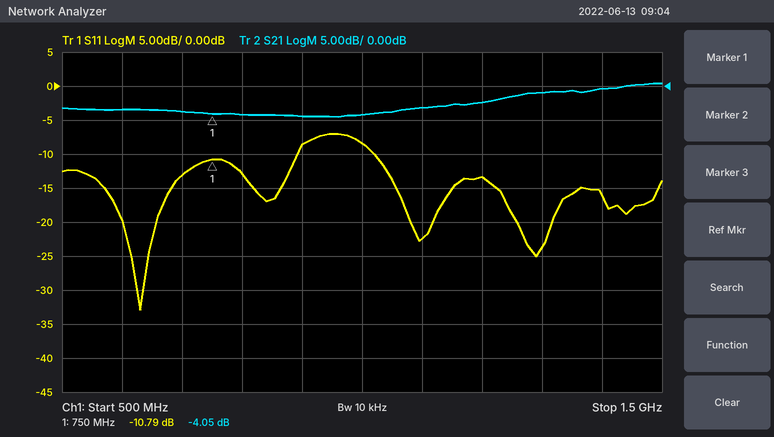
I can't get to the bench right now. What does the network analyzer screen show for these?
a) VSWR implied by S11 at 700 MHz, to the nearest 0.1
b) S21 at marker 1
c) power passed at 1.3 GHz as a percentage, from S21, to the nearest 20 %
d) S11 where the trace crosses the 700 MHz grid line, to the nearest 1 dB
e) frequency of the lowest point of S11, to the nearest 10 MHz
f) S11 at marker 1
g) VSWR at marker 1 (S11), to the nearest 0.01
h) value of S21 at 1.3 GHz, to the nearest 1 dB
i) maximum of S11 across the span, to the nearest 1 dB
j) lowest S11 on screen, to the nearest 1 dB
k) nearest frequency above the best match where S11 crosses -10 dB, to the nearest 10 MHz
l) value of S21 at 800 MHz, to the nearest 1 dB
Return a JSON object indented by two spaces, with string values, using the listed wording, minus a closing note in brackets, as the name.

{
  "VSWR implied by S11 at 700 MHz, to the nearest 0.1": "1.6",
  "S21 at marker 1": "-4.05 dB",
  "power passed at 1.3 GHz as a percentage, from S21, to the nearest 20 %": "80 %",
  "S11 where the trace crosses the 700 MHz grid line, to the nearest 1 dB": "-13 dB",
  "frequency of the lowest point of S11, to the nearest 10 MHz": "630 MHz",
  "S11 at marker 1": "-10.79 dB",
  "VSWR at marker 1 (S11), to the nearest 0.01": "1.81",
  "value of S21 at 1.3 GHz, to the nearest 1 dB": "-1 dB",
  "maximum of S11 across the span, to the nearest 1 dB": "-7 dB",
  "lowest S11 on screen, to the nearest 1 dB": "-33 dB",
  "nearest frequency above the best match where S11 crosses -10 dB, to the nearest 10 MHz": "890 MHz",
  "value of S21 at 800 MHz, to the nearest 1 dB": "-4 dB"
}
